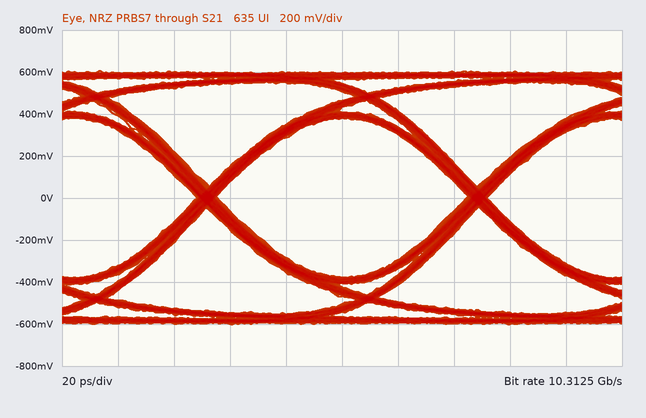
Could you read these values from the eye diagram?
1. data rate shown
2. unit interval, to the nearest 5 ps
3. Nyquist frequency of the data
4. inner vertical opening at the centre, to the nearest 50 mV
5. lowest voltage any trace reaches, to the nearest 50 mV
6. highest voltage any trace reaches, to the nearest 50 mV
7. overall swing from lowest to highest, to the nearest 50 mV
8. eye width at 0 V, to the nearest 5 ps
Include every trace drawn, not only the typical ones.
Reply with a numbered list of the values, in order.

1. 10.3125 Gb/s
2. 95 ps
3. 5.15625 GHz
4. 750 mV
5. -600 mV
6. 600 mV
7. 1.20 V
8. 90 ps
